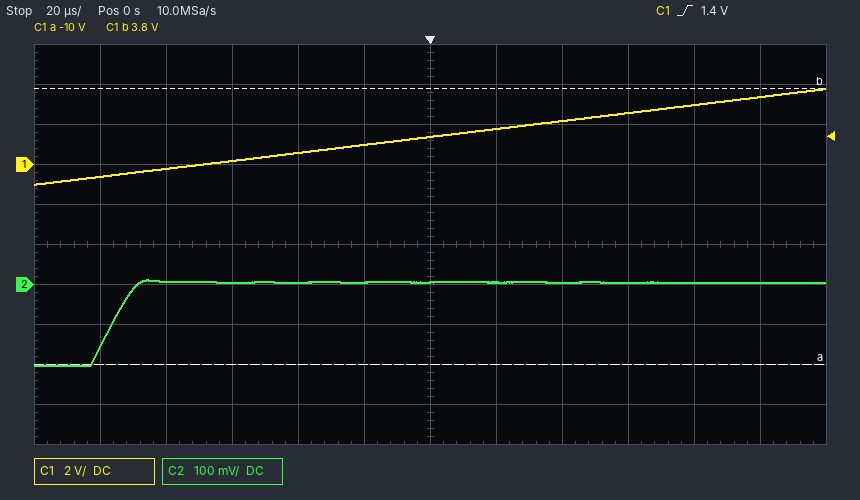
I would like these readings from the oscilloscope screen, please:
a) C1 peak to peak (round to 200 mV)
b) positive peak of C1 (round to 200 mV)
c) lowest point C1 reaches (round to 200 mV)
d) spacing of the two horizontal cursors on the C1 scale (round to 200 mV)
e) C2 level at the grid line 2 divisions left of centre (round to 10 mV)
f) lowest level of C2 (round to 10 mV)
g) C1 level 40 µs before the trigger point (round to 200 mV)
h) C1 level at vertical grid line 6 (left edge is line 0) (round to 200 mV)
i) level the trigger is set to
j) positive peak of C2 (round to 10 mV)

4.8 V
3.8 V
-1.0 V
13.8 V
10 mV
-200 mV
600 mV
1.4 V
1.4 V
10 mV
